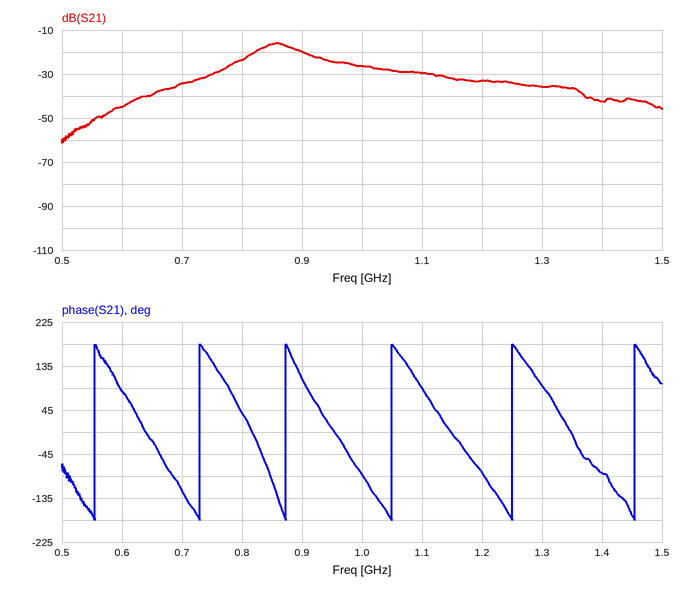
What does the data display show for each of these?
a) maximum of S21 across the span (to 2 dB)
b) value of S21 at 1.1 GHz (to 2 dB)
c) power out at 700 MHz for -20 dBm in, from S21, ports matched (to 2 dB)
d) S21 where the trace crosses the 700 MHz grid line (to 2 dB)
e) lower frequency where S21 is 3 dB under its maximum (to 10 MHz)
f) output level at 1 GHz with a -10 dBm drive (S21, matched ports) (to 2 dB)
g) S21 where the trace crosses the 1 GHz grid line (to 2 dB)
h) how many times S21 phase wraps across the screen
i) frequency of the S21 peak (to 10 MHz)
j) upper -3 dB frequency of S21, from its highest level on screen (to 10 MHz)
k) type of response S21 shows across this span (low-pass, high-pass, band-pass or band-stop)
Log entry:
-16 dB
-30 dB
-54 dBm
-34 dB
830 MHz
-36 dBm
-26 dB
6
860 MHz
890 MHz
band-pass
